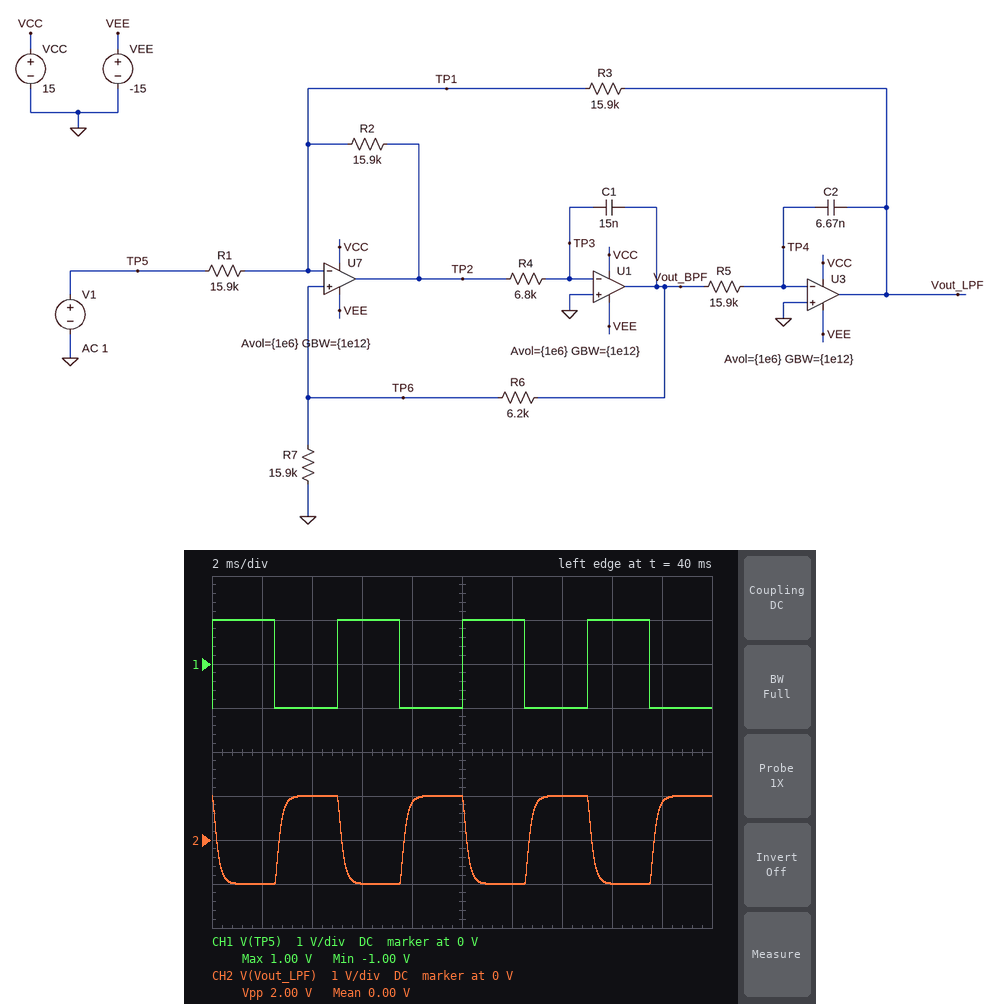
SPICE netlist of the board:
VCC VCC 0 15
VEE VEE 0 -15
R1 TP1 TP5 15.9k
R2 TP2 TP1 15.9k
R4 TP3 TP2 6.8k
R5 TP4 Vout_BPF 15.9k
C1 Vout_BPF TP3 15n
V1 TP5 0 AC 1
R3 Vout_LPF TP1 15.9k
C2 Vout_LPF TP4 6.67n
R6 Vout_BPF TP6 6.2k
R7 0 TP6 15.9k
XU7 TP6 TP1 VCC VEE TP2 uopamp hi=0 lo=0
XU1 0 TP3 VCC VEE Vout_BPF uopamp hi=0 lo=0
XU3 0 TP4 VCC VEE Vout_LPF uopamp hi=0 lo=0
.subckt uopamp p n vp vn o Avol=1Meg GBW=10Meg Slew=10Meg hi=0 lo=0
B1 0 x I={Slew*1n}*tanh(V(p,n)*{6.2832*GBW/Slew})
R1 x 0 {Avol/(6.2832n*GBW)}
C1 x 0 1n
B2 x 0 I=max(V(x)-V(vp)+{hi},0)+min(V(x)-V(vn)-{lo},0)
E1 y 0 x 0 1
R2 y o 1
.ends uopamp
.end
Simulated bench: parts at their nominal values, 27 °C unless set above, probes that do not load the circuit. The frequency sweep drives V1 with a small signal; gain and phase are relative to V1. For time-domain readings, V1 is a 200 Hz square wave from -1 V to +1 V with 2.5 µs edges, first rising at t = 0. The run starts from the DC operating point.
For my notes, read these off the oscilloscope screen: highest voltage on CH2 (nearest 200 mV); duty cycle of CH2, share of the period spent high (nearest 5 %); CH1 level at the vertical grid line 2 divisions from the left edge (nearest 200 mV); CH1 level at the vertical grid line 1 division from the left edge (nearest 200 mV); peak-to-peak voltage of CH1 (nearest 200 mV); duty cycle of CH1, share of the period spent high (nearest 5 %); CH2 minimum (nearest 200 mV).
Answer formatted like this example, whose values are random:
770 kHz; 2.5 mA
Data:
1.0 V; 50 %; -1.0 V; 1.0 V; 2.0 V; 50 %; -1.0 V
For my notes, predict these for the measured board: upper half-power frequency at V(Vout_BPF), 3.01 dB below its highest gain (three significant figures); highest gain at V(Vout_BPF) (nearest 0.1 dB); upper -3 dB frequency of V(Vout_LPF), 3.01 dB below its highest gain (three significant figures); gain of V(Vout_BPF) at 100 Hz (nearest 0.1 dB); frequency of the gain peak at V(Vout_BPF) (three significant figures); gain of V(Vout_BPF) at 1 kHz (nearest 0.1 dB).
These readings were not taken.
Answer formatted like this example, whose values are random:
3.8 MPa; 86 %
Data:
3.96 kHz; -6.7 dB; 861 Hz; -23.6 dB; 1.53 kHz; -7.3 dB
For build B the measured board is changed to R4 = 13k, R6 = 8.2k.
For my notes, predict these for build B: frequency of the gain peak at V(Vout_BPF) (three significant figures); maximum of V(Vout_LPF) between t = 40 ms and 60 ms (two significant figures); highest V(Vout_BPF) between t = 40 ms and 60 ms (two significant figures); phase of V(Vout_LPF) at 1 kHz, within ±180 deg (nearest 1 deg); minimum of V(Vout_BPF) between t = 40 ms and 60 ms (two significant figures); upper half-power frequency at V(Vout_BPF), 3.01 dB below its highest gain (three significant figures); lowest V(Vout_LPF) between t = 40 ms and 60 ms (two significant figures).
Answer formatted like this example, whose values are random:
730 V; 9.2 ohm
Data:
1.11 kHz; 1.1 V; 660 mV; 98 deg; -660 mV; 2.18 kHz; -1.1 V
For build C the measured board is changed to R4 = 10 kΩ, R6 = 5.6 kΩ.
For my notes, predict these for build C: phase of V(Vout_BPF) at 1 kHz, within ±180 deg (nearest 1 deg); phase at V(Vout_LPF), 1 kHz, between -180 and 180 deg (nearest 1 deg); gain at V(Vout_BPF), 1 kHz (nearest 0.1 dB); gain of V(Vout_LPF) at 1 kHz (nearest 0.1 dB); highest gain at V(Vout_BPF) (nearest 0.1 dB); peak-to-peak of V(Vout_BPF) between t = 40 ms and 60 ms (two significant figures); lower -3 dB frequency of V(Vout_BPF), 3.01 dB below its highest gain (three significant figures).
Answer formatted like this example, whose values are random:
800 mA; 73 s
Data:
14 deg; 104 deg; -7.2 dB; -3.7 dB; -6.9 dB; 1.3 V; 549 Hz
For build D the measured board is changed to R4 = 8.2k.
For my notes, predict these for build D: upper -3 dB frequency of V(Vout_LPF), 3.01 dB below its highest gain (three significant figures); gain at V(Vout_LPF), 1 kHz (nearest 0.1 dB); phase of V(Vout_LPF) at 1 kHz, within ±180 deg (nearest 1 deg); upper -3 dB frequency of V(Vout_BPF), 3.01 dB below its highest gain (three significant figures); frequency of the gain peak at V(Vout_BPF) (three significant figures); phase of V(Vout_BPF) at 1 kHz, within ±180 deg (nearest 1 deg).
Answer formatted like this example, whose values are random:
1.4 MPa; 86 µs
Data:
894 Hz; -3.6 dB; 109 deg; 3.37 kHz; 1.39 kHz; 19 deg
